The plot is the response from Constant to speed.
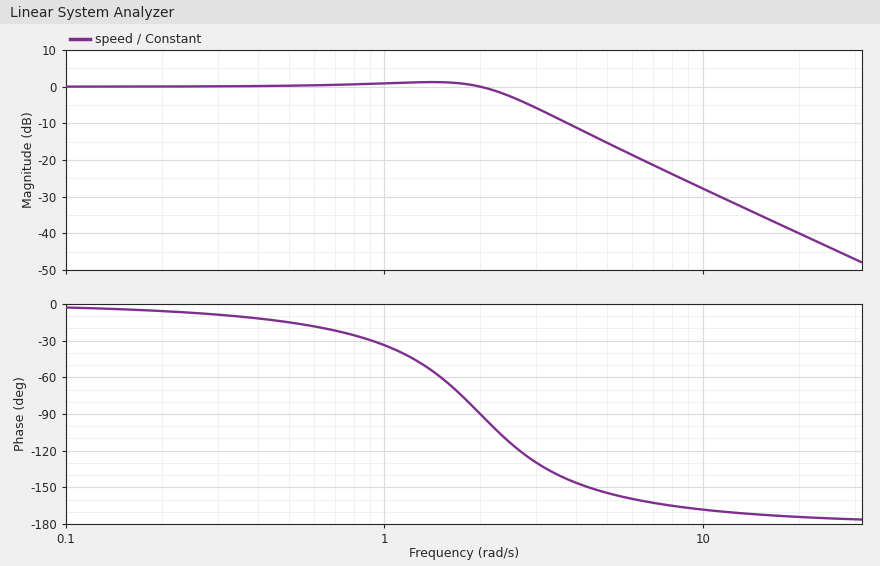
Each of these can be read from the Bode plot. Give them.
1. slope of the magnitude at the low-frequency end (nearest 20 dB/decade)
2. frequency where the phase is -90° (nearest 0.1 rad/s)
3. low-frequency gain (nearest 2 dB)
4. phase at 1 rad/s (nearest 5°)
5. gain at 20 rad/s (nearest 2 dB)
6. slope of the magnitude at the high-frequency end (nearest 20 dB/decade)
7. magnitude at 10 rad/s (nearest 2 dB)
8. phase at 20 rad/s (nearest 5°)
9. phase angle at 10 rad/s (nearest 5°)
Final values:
0 dB/decade
2.0 rad/s
0 dB
-35°
-40 dB
-40 dB/decade
-28 dB
-175°
-170°
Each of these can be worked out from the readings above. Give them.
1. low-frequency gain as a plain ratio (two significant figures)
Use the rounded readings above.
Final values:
1.0
